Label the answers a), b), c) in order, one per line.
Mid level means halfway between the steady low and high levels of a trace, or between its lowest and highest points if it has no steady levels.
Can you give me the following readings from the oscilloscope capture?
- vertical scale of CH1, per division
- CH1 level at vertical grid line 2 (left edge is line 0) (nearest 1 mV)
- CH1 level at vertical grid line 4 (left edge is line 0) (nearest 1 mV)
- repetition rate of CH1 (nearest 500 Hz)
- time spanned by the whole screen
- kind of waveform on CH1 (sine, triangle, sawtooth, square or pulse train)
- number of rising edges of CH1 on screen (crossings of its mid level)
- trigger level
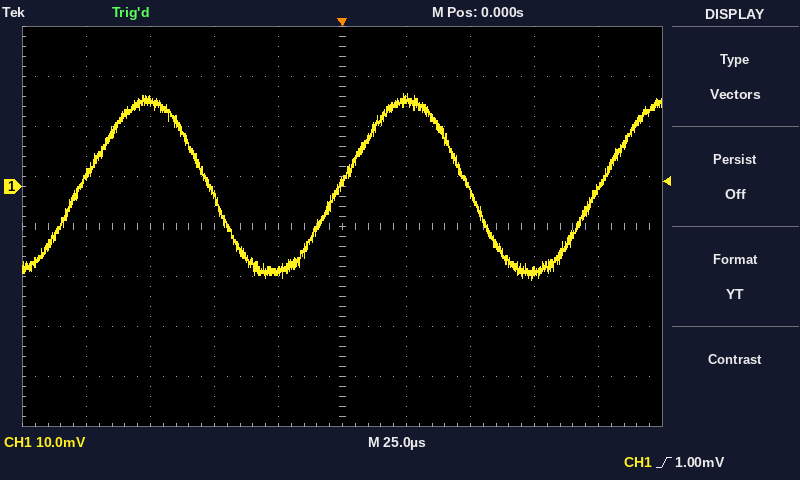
a) 10 mV
b) 17 mV
c) -17 mV
d) 10.0 kHz
e) 250 µs
f) sine
g) 3
h) 1.00 mV
